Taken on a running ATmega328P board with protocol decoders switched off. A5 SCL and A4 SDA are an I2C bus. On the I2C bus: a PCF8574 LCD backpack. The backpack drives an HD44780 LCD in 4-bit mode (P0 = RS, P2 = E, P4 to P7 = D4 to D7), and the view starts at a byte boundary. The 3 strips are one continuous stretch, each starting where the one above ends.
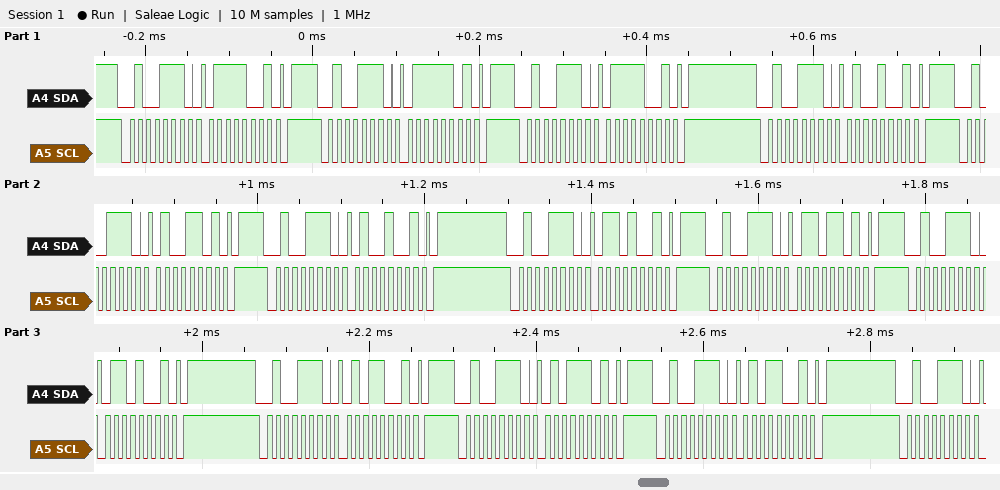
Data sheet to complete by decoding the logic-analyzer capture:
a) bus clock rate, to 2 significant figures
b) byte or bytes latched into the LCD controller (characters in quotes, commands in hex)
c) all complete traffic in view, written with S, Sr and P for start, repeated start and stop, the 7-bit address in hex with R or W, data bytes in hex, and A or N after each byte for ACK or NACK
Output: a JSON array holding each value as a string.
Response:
["100 kHz", "'t' 'e'", "S 27W A 79 A P S 27W A 7D A P S 27W A 79 A P S 27W A 49 A P S 27W A 4D A P S 27W A 49 A P S 27W A 69 A P S 27W A 6D A P S 27W A 69 A P S 27W A 59 A P S 27W A 5D A P S 27W A 59 A P S 27W A"]
